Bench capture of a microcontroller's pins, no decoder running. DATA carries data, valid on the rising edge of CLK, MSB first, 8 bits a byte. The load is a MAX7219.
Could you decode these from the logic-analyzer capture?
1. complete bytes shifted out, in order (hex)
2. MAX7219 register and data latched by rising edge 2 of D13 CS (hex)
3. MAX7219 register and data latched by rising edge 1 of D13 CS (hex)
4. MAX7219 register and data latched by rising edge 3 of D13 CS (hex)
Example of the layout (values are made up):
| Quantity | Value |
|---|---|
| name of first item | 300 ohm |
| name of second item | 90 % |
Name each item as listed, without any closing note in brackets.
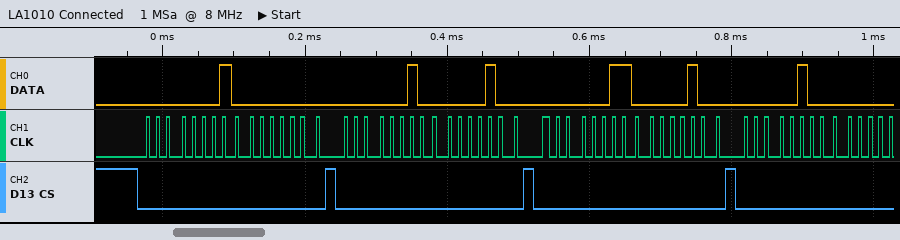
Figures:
| Quantity | Value |
|---|---|
| complete bytes shifted out, in order | 01 00 02 04 03 04 04 |
| MAX7219 register and data latched by rising edge 2 of D13 CS | register 0x2, data 0x04 |
| MAX7219 register and data latched by rising edge 1 of D13 CS | register 0x1, data 0x00 |
| MAX7219 register and data latched by rising edge 3 of D13 CS | register 0x3, data 0x04 |
